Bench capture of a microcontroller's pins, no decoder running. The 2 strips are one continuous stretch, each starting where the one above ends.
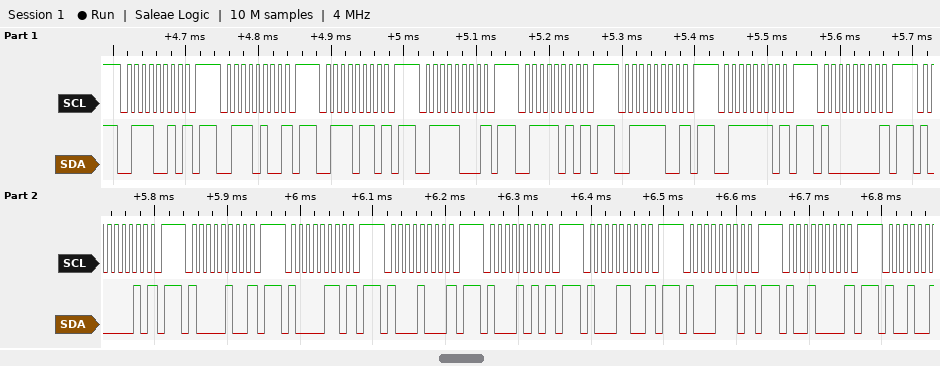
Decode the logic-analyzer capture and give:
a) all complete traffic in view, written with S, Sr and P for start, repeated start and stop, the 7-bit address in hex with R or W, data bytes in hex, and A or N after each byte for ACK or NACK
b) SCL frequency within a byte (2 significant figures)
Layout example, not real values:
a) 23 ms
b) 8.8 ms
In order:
a) S 39W N P S 3AW N P S 3BW N P S 3CW N P S 3DW N P S 3EW N P S 3FW N P S 40W N P S 41W N P S 42W N P S 43W N P S 44W N P S 45W N P S 46W N P S 47W N P S 48W N P
b) 100 kHz
